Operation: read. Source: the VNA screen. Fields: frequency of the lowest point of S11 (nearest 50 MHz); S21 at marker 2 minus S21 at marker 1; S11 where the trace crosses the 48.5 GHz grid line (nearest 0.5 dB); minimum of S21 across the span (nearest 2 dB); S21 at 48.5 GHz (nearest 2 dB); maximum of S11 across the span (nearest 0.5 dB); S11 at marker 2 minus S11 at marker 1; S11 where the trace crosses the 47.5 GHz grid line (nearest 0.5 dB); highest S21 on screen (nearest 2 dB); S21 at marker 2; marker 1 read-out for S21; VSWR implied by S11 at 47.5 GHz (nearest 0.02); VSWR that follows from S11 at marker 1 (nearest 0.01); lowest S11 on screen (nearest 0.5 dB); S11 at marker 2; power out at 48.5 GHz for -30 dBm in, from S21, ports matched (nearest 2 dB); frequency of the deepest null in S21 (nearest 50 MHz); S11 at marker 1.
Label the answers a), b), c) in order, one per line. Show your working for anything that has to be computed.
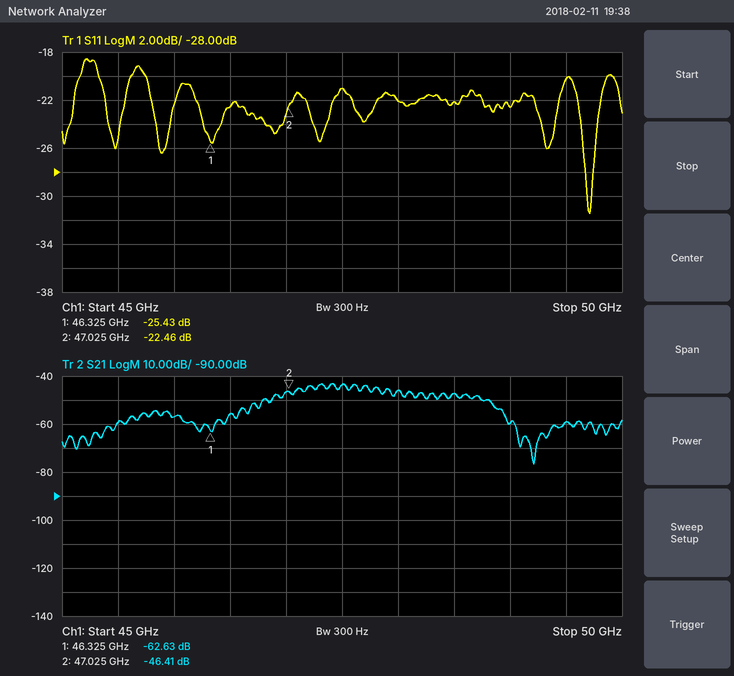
a) 49.70 GHz
b) -46.41 − (-62.63) = 16.22 dB
c) -22.0 dB
d) -76 dB
e) -48 dB
f) -18.5 dB
g) -22.46 − (-25.43) = 2.97 dB
h) -21.0 dB
i) -44 dB
j) -46.41 dB
k) -62.63 dB
l) |Γ| = 10^(-21/20) = 0.0891; VSWR = (1 + 0.0891)/(1 − 0.0891) ≈ 1.20
m) (1 + 0.0535)/(1 − 0.0535) ≈ 1.11
n) -31.5 dB
o) -22.46 dB
p) -30 dBm + (-48 dB) = -78 dBm
q) 49.20 GHz
r) -25.43 dB
